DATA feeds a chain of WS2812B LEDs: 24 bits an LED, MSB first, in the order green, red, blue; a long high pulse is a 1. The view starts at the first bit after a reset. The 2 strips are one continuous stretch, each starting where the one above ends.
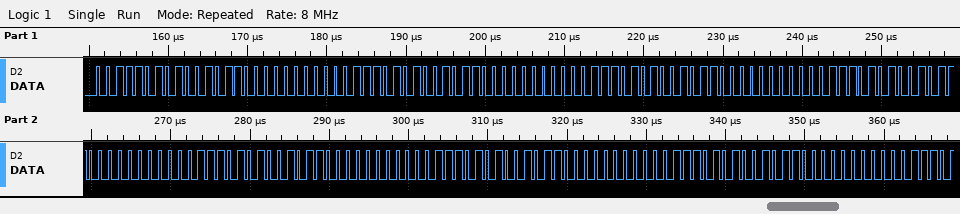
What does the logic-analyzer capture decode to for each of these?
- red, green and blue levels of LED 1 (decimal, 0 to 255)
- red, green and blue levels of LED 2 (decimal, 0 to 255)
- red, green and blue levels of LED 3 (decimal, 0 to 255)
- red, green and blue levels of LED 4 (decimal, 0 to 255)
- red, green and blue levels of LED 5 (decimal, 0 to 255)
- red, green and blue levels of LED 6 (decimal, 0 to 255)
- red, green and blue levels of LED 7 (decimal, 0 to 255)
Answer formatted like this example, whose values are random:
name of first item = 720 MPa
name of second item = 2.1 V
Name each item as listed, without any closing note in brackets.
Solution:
red, green and blue levels of LED 1 = 150, 58, 0
red, green and blue levels of LED 2 = 150, 58, 0
red, green and blue levels of LED 3 = 150, 58, 0
red, green and blue levels of LED 4 = 150, 58, 0
red, green and blue levels of LED 5 = 150, 58, 0
red, green and blue levels of LED 6 = 150, 58, 0
red, green and blue levels of LED 7 = 150, 58, 0
